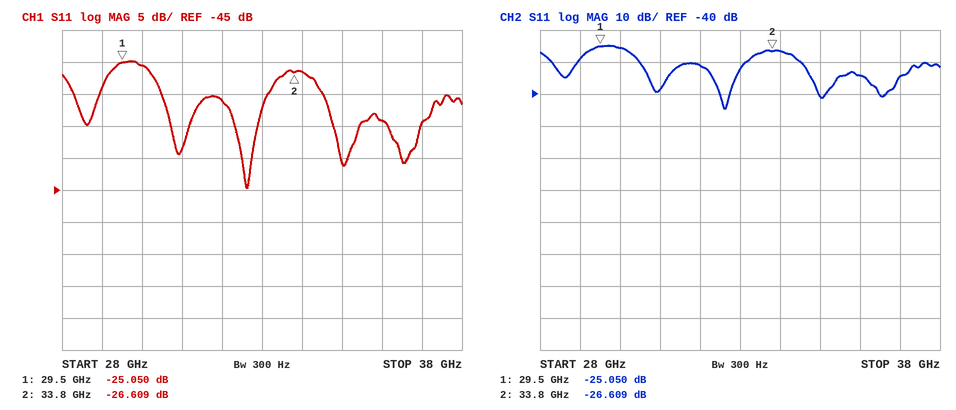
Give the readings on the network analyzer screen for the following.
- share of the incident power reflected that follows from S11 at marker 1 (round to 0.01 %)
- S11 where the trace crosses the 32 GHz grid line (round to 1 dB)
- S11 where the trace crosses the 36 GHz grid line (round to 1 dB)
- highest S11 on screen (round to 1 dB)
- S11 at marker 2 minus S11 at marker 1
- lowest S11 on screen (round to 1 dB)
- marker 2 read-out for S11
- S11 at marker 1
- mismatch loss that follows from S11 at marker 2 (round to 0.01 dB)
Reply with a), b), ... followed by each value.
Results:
a) 0.31 %
b) -31 dB
c) -34 dB
d) -25 dB
e) -1.559 dB
f) -45 dB
g) -26.609 dB
h) -25.050 dB
i) 0.01 dB
